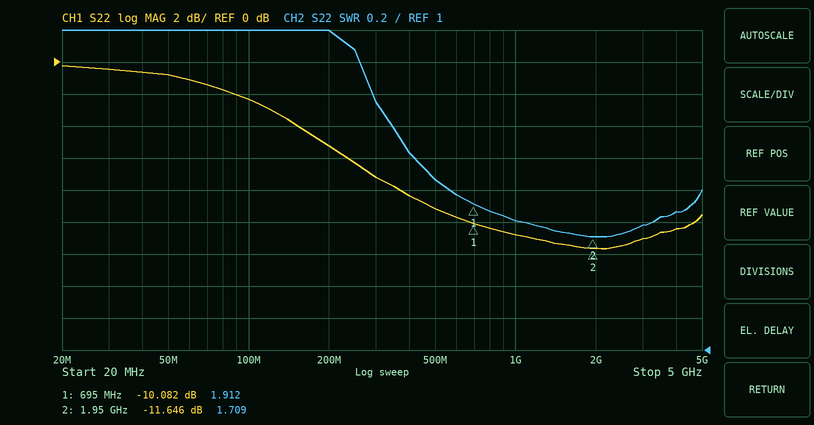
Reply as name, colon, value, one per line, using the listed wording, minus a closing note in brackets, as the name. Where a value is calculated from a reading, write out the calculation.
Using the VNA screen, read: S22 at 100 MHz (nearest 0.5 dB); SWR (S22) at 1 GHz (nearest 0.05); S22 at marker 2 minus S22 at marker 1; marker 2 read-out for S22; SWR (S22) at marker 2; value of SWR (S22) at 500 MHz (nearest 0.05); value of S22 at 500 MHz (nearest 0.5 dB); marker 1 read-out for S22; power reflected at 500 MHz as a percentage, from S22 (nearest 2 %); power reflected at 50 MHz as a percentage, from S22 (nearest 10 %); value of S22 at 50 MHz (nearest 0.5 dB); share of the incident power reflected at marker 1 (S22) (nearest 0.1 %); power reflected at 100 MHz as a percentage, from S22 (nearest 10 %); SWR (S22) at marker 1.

S22 at 100 MHz: -2.5 dB
SWR (S22) at 1 GHz: 1.80
S22 at marker 2 minus S22 at marker 1: -11.646 − (-10.082) = -1.564 dB
marker 2 read-out for S22: -11.646 dB
SWR (S22) at marker 2: 1.709
value of SWR (S22) at 500 MHz: 2.05
value of S22 at 500 MHz: -9.0 dB
marker 1 read-out for S22: -10.082 dB
power reflected at 500 MHz as a percentage, from S22: 10^(-9/10) ≈ 12.6 %, so 12 % to the nearest 2 %
power reflected at 50 MHz as a percentage, from S22: 10^(-1/10) ≈ 79.4 %, so 80 % to the nearest 10 %
value of S22 at 50 MHz: -1.0 dB
share of the incident power reflected at marker 1 (S22): 10^(-10.082/10) ≈ 9.8 %
power reflected at 100 MHz as a percentage, from S22: 10^(-2.5/10) ≈ 56.2 %, so 60 % to the nearest 10 %
SWR (S22) at marker 1: 1.912
